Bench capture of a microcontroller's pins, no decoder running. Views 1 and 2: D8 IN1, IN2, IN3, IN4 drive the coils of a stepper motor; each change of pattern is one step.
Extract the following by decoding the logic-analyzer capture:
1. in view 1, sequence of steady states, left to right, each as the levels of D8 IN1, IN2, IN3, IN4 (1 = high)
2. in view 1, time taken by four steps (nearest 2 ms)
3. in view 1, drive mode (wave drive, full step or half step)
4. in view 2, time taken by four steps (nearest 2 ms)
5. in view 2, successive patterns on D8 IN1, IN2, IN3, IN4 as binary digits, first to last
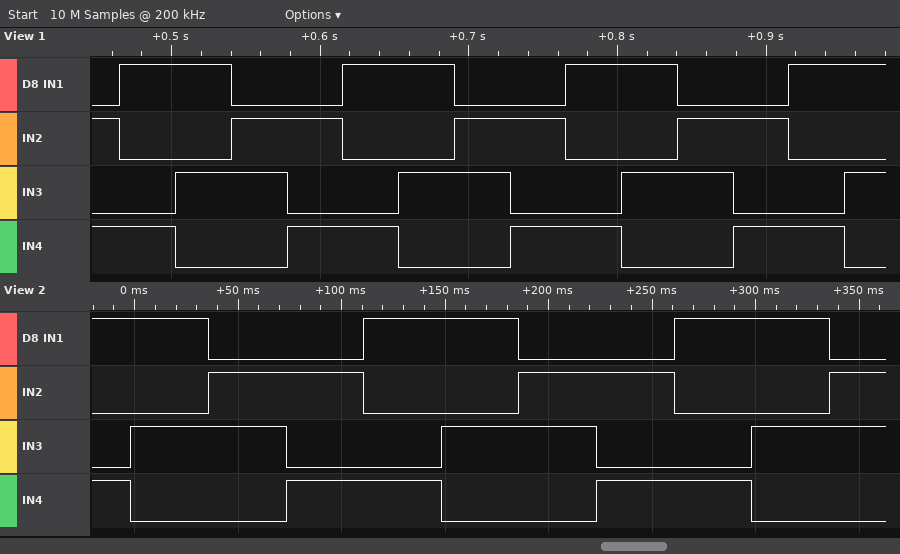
0101 1001 1010 0110 0101 1001 1010 0110 0101 1001 1010 0110 0101 1001 1010
150 ms
full step
150 ms
1001 1010 0110 0101 1001 1010 0110 0101 1001 1010 0110
